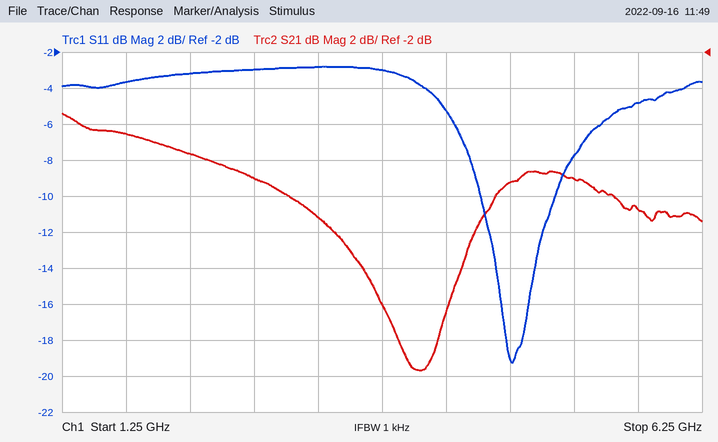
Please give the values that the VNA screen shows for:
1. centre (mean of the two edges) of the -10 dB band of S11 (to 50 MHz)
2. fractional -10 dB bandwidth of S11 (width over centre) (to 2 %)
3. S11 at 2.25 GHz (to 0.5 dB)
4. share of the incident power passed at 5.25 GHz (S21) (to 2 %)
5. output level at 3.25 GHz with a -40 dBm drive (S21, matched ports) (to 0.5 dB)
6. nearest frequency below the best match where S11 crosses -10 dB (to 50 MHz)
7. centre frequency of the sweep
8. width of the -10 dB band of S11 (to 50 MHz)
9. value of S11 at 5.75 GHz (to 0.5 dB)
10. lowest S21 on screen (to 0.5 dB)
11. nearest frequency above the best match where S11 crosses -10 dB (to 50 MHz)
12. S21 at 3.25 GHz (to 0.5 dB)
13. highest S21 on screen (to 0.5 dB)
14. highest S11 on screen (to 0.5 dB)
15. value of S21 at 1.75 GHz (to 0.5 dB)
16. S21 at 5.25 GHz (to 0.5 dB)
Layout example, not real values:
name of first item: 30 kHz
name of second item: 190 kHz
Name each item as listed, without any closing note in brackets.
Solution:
centre (mean of the two edges) of the -10 dB band of S11: 4.80 GHz
fractional -10 dB bandwidth of S11 (width over centre): 12 %
S11 at 2.25 GHz: -3.0 dB
share of the incident power passed at 5.25 GHz (S21): 12 %
output level at 3.25 GHz with a -40 dBm drive (S21, matched ports): -51.0 dBm
nearest frequency below the best match where S11 crosses -10 dB: 4.50 GHz
centre frequency of the sweep: 3.75 GHz
width of the -10 dB band of S11: 600 MHz
value of S11 at 5.75 GHz: -5.0 dB
lowest S21 on screen: -19.5 dB
nearest frequency above the best match where S11 crosses -10 dB: 5.10 GHz
S21 at 3.25 GHz: -11.0 dB
highest S21 on screen: -5.5 dB
highest S11 on screen: -3.0 dB
value of S21 at 1.75 GHz: -6.5 dB
S21 at 5.25 GHz: -9.0 dB
